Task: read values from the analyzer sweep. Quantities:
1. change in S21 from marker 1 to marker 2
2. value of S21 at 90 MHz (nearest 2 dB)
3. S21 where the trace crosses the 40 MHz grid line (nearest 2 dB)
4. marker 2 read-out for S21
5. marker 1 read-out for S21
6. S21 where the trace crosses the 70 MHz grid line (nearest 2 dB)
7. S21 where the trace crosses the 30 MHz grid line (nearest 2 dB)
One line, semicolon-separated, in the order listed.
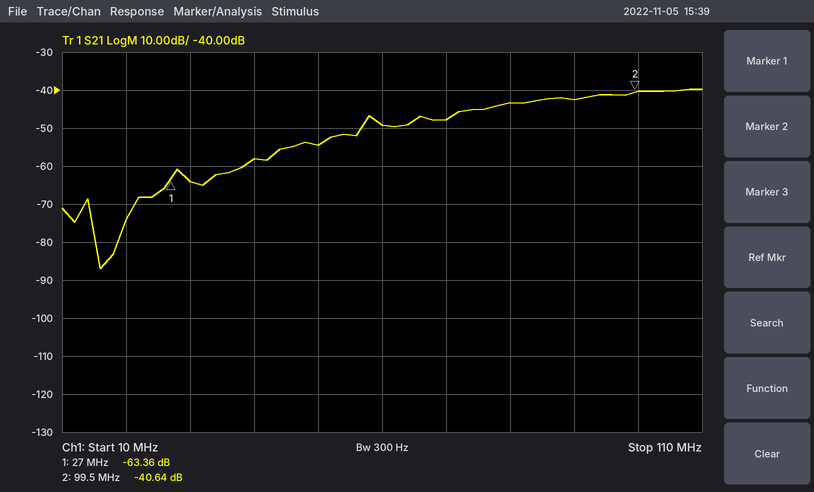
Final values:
22.72 dB; -42 dB; -58 dB; -40.64 dB; -63.36 dB; -48 dB; -64 dB
